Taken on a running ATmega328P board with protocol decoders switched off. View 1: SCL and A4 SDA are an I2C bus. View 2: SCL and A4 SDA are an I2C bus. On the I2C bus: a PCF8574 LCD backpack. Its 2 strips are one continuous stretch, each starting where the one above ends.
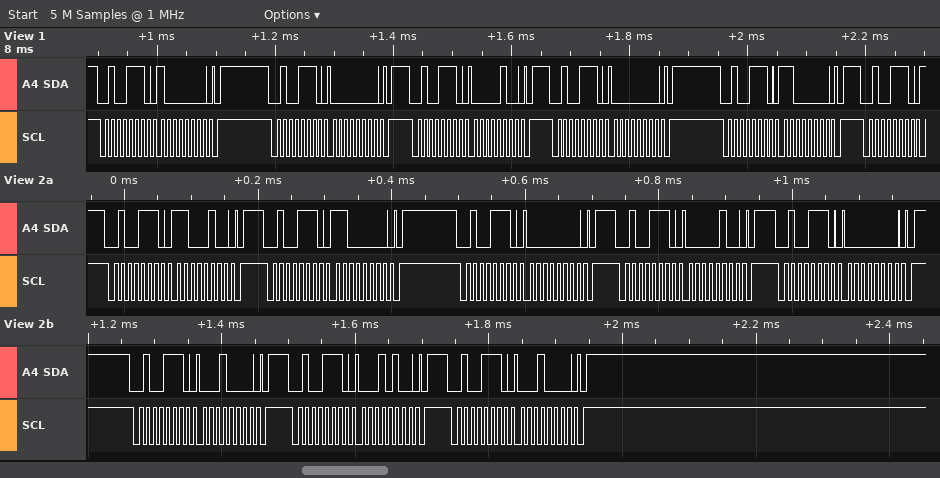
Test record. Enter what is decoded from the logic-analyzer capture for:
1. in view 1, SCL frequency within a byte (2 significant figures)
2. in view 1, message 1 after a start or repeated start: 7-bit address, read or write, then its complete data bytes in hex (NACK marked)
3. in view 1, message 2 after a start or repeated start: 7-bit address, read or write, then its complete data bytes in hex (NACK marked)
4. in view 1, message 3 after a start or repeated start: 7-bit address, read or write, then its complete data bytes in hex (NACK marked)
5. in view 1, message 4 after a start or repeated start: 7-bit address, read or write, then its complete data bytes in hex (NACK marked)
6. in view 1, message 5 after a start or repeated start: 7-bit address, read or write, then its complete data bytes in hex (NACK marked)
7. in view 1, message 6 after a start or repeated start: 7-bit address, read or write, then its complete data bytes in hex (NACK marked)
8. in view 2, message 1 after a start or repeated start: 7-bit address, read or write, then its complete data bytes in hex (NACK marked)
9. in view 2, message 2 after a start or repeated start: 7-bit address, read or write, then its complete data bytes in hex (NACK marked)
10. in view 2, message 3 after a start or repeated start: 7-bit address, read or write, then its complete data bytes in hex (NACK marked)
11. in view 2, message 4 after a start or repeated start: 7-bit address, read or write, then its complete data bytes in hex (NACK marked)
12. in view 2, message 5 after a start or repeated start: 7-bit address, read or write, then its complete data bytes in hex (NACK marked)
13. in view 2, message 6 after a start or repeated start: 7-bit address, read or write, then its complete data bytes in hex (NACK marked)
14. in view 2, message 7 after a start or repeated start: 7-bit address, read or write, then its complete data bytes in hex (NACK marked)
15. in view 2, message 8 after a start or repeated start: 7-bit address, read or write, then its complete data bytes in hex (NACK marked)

100 kHz
0x27 write: 80
0x27 write: 00
0x27 write: 04
0x27 write: 00
0x27 write: C0
0x27 write
0x27 write: C4
0x27 write: C0
0x27 write: 00
0x27 write: 04
0x27 write: 00
0x27 write: 10
0x27 write: 14
0x27 write: 10
